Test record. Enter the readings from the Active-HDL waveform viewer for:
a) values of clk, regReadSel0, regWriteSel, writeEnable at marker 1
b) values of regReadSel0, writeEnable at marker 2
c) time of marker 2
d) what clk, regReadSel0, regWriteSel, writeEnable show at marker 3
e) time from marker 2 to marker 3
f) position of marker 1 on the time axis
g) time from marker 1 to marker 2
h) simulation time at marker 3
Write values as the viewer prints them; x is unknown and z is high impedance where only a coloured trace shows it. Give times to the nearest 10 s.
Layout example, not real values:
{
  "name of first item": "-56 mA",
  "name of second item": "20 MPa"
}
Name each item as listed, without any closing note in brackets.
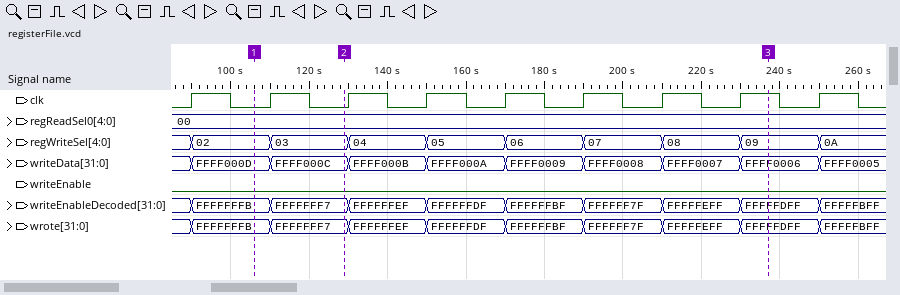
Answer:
{
  "values of clk, regReadSel0, regWriteSel, writeEnable at marker 1": "clk=0, regReadSel0=00, regWriteSel=02, writeEnable=0",
  "values of regReadSel0, writeEnable at marker 2": "regReadSel0=00, writeEnable=0",
  "time of marker 2": "130 s",
  "what clk, regReadSel0, regWriteSel, writeEnable show at marker 3": "clk=1, regReadSel0=00, regWriteSel=09, writeEnable=0",
  "time from marker 2 to marker 3": "110 s",
  "position of marker 1 on the time axis": "110 s",
  "time from marker 1 to marker 2": "20 s",
  "simulation time at marker 3": "240 s"
}
